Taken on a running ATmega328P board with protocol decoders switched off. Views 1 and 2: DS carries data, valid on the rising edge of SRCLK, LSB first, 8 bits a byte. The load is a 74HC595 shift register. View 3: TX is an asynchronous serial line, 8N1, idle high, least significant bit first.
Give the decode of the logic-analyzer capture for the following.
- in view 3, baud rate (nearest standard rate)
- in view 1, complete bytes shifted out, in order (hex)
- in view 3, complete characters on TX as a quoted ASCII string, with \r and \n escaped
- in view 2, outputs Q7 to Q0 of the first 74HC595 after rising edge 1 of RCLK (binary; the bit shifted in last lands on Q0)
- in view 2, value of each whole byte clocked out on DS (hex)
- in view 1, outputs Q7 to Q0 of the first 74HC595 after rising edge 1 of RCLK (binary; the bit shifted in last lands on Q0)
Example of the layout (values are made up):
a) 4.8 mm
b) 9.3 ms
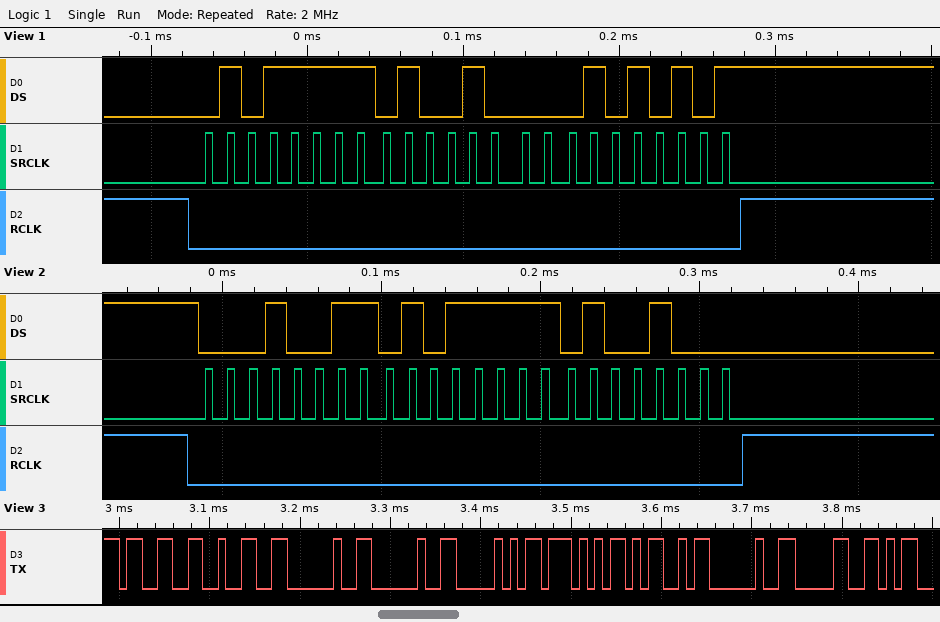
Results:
a) 115200 baud
b) FA 12 AA
c) "32  PWM 0"
d) 01001000
e) C8 FA 12
f) 01010101
